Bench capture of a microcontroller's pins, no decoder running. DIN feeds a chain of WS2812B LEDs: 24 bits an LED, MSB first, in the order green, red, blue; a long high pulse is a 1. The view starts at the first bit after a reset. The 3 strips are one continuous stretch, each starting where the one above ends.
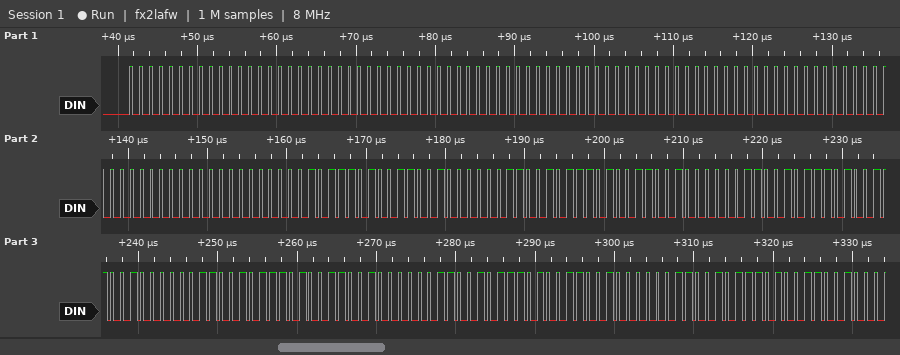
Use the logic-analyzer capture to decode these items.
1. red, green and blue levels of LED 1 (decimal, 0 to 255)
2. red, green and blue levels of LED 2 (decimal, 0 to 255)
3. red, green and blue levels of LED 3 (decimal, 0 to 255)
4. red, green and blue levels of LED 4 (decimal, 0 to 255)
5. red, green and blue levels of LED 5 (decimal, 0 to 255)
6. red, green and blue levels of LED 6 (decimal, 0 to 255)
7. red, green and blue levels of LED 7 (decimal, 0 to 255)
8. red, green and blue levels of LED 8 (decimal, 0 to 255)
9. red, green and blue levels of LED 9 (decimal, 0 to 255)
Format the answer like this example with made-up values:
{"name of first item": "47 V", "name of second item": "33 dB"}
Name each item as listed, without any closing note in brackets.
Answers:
{"red, green and blue levels of LED 1": "0, 0, 0", "red, green and blue levels of LED 2": "0, 0, 0", "red, green and blue levels of LED 3": "0, 0, 0", "red, green and blue levels of LED 4": "0, 0, 0", "red, green and blue levels of LED 5": "50, 93, 6", "red, green and blue levels of LED 6": "50, 93, 6", "red, green and blue levels of LED 7": "50, 93, 6", "red, green and blue levels of LED 8": "50, 93, 6", "red, green and blue levels of LED 9": "50, 93, 6"}
